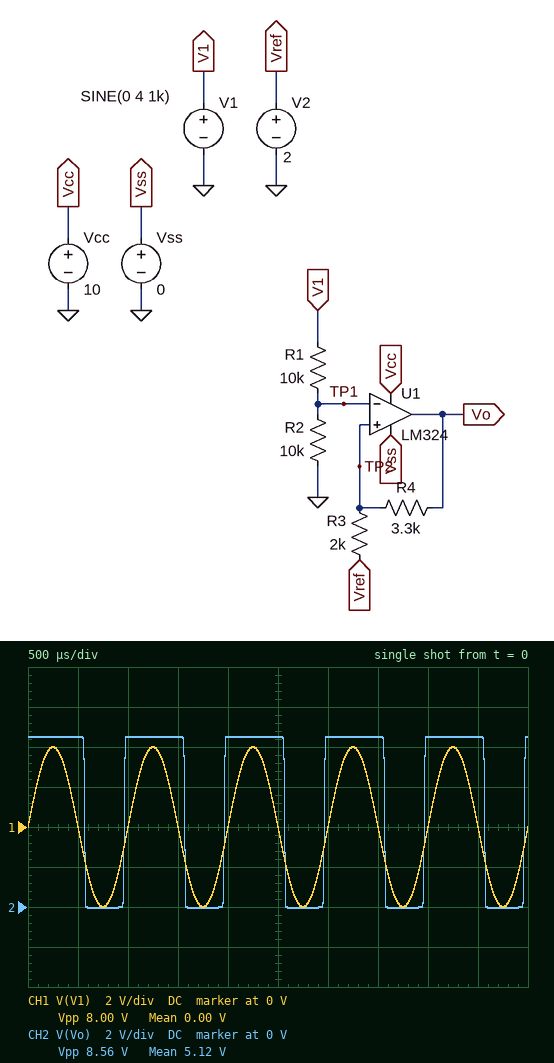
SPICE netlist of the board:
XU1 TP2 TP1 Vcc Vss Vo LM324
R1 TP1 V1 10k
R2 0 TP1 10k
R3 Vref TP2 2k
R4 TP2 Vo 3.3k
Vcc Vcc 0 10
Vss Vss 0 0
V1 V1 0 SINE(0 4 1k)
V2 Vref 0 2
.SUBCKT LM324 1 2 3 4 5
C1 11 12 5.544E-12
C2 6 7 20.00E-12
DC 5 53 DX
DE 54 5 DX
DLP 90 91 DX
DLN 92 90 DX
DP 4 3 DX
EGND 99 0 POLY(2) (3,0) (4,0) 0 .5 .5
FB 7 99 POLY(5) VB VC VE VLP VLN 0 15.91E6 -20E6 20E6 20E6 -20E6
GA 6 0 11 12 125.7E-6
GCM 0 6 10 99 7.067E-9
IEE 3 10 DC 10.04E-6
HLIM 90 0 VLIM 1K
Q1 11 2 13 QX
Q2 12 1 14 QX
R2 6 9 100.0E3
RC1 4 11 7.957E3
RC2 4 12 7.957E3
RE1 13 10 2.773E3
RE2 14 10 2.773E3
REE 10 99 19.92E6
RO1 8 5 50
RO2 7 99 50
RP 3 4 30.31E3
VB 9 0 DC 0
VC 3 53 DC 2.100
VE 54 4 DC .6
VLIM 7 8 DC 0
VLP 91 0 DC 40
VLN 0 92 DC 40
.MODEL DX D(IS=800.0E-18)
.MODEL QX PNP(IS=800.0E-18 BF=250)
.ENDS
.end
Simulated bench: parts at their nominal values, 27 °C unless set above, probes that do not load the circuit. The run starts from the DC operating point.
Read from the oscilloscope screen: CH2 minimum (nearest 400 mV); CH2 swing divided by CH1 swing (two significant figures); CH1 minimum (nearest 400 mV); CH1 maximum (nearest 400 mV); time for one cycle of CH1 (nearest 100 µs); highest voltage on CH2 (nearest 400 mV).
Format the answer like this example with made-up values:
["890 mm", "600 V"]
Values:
["0 V", "1.1", "-4.0 V", "4.0 V", "1.0 ms", "8.4 V"]
